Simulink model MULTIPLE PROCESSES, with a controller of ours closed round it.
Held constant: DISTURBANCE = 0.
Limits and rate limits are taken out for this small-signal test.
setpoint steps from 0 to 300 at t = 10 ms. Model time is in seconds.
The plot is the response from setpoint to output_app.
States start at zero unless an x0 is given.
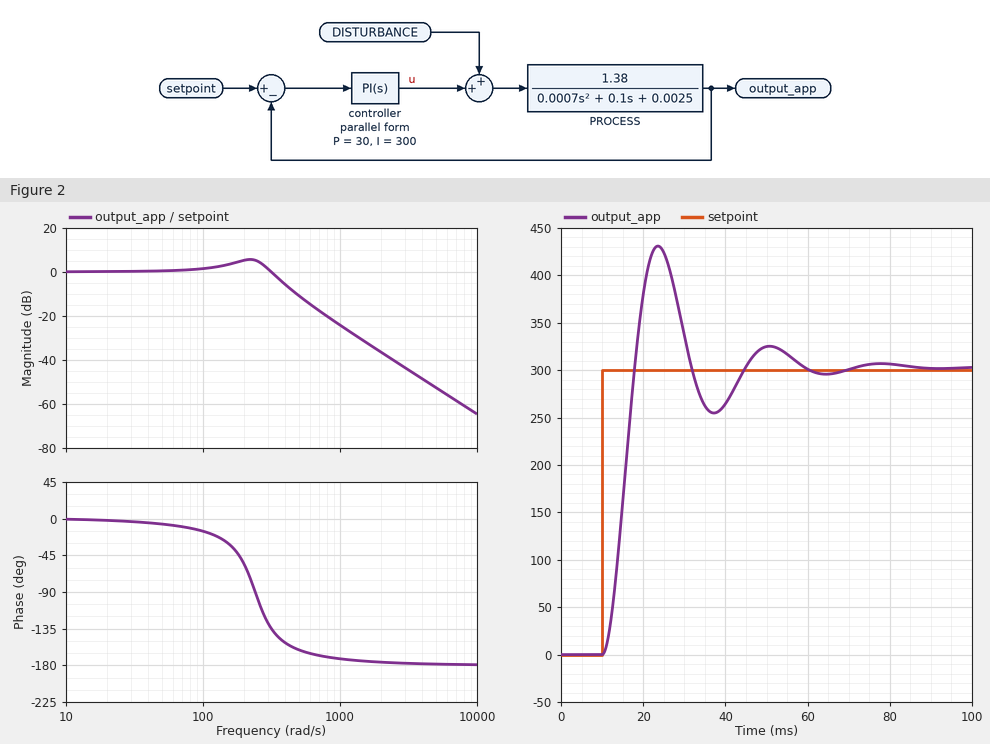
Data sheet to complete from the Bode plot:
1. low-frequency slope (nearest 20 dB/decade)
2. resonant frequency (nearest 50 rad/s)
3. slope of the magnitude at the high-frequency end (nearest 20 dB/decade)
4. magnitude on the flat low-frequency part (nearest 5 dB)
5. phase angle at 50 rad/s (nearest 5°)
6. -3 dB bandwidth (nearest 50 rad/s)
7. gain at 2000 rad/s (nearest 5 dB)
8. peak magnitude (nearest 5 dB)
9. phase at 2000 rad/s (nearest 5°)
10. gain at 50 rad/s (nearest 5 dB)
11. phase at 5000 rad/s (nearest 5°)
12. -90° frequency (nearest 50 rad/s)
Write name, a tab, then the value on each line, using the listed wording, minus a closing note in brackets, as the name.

low-frequency slope	0 dB/decade
resonant frequency	200 rad/s
slope of the magnitude at the high-frequency end	-40 dB/decade
magnitude on the flat low-frequency part	0 dB
phase angle at 50 rad/s	-5°
-3 dB bandwidth	350 rad/s
gain at 2000 rad/s	-35 dB
peak magnitude	5 dB
phase at 2000 rad/s	-175°
gain at 50 rad/s	0 dB
phase at 5000 rad/s	-180°
-90° frequency	250 rad/s
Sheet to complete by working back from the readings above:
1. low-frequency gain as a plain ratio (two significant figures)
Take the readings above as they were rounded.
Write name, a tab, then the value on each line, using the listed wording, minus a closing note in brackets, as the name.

low-frequency gain as a plain ratio	1.0
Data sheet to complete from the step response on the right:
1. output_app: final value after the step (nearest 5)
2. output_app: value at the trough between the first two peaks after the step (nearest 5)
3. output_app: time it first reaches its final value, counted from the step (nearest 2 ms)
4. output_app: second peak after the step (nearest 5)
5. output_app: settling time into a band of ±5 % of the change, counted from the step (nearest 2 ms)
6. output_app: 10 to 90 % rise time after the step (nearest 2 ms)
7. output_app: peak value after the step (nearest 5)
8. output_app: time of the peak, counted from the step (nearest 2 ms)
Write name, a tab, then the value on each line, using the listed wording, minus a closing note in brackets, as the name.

output_app: final value after the step	300
output_app: value at the trough between the first two peaks after the step	255
output_app: time it first reaches its final value, counted from the step	8 ms
output_app: second peak after the step	325
output_app: settling time into a band of ±5 % of the change, counted from the step	46 ms
output_app: 10 to 90 % rise time after the step	6 ms
output_app: peak value after the step	430
output_app: time of the peak, counted from the step	14 ms
